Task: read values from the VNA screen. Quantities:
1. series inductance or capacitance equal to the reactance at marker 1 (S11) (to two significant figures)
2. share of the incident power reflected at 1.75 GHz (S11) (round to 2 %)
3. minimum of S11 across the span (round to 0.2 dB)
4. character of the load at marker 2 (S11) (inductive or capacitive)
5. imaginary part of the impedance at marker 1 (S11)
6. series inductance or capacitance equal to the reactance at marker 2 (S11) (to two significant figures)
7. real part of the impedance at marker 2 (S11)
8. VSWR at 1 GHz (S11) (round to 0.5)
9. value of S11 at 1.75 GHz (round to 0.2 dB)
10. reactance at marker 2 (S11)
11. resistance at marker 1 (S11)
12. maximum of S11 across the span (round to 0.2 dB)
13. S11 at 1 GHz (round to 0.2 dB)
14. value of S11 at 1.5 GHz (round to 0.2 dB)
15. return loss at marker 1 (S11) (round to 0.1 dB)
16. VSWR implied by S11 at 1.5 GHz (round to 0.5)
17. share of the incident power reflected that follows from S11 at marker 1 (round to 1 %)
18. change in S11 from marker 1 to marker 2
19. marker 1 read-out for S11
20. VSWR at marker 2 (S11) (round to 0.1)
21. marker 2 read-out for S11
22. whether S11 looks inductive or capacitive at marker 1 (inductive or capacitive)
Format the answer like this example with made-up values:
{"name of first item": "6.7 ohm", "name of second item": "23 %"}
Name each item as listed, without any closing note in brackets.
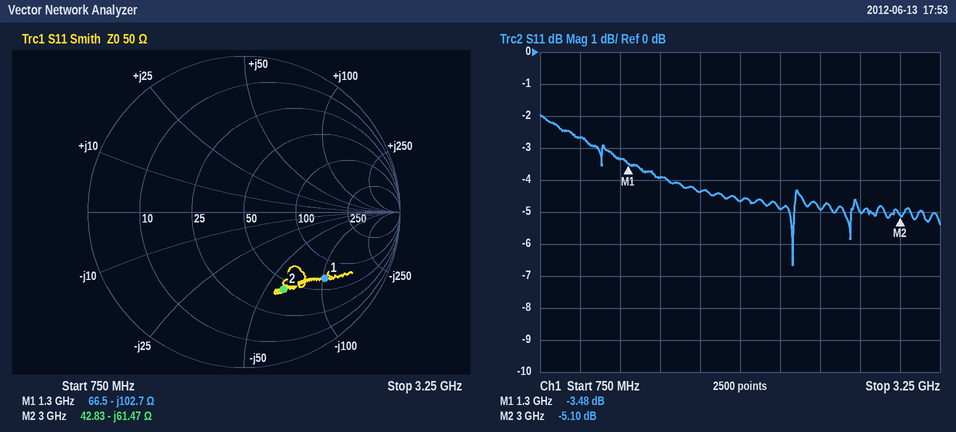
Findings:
{"series inductance or capacitance equal to the reactance at marker 1 (S11)": "1.2 pF", "share of the incident power reflected at 1.75 GHz (S11)": "36 %", "minimum of S11 across the span": "-6.6 dB", "character of the load at marker 2 (S11)": "capacitive", "imaginary part of the impedance at marker 1": "-102.7 Ω", "series inductance or capacitance equal to the reactance at marker 2 (S11)": "860 fF", "real part of the impedance at marker 2": "42.83 Ω", "VSWR at 1 GHz (S11)": "6.5", "value of S11 at 1.75 GHz": "-4.4 dB", "reactance at marker 2": "-61.47 Ω", "resistance at marker 1": "66.5 Ω", "maximum of S11 across the span": "-2.0 dB", "S11 at 1 GHz": "-2.6 dB", "value of S11 at 1.5 GHz": "-4.0 dB", "return loss at marker 1 (S11)": "3.5 dB", "VSWR implied by S11 at 1.5 GHz": "4.5", "share of the incident power reflected that follows from S11 at marker 1": "45 %", "change in S11 from marker 1 to marker 2": "-1.62 dB", "marker 1 read-out for S11": "-3.48 dB", "VSWR at marker 2 (S11)": "3.5", "marker 2 read-out for S11": "-5.10 dB", "whether S11 looks inductive or capacitive at marker 1": "capacitive"}
